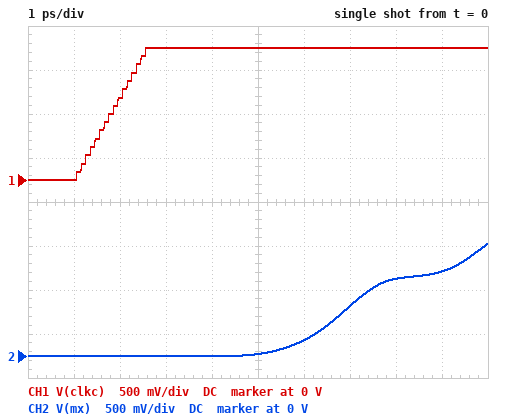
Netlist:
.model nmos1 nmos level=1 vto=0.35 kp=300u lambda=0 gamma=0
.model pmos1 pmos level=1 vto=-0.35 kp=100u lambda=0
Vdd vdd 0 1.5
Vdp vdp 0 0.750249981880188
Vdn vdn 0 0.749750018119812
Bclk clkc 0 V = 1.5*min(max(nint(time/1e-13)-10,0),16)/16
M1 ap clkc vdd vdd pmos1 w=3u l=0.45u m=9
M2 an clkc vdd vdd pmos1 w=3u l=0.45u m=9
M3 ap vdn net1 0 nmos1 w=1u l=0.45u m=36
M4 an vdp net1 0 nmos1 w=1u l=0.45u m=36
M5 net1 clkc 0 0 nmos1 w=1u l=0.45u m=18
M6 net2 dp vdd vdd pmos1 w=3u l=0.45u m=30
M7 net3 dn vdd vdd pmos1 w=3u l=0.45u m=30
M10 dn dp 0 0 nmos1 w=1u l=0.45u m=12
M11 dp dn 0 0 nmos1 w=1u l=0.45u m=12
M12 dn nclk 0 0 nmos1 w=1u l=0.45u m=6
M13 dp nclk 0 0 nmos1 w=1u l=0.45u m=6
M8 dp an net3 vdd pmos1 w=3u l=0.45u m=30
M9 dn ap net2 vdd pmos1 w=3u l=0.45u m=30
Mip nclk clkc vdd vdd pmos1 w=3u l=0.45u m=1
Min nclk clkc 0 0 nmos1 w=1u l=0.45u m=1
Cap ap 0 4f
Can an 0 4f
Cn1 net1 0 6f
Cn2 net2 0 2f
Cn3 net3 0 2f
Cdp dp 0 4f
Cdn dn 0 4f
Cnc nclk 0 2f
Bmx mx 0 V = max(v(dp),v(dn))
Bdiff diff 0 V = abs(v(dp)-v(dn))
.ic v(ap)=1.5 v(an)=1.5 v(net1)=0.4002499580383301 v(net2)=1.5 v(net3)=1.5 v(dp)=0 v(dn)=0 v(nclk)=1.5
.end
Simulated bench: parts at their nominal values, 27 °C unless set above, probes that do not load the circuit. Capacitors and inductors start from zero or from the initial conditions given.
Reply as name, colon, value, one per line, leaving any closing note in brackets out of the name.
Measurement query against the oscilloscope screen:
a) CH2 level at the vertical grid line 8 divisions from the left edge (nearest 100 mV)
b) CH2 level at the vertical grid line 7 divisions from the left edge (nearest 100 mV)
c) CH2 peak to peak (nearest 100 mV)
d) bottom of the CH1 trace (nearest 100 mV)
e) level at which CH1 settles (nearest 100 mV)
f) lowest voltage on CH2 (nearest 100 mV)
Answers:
CH2 level at the vertical grid line 8 divisions from the left edge: 900 mV
CH2 level at the vertical grid line 7 divisions from the left edge: 600 mV
CH2 peak to peak: 1.3 V
bottom of the CH1 trace: 0 V
level at which CH1 settles: 1.5 V
lowest voltage on CH2: 0 V
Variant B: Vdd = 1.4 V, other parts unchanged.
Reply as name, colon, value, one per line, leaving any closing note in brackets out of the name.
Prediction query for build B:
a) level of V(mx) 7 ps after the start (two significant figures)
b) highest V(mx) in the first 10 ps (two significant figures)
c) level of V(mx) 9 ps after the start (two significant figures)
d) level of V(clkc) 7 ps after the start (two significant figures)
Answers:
level of V(mx) 7 ps after the start: 540 mV
highest V(mx) in the first 10 ps: 1.1 V
level of V(mx) 9 ps after the start: 860 mV
level of V(clkc) 7 ps after the start: 1.5 V
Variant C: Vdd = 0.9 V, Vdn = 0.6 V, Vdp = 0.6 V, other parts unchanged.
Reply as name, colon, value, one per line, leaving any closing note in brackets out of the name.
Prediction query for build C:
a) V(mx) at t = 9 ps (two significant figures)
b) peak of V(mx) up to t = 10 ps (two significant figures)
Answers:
V(mx) at t = 9 ps: 29 mV
peak of V(mx) up to t = 10 ps: 110 mV
